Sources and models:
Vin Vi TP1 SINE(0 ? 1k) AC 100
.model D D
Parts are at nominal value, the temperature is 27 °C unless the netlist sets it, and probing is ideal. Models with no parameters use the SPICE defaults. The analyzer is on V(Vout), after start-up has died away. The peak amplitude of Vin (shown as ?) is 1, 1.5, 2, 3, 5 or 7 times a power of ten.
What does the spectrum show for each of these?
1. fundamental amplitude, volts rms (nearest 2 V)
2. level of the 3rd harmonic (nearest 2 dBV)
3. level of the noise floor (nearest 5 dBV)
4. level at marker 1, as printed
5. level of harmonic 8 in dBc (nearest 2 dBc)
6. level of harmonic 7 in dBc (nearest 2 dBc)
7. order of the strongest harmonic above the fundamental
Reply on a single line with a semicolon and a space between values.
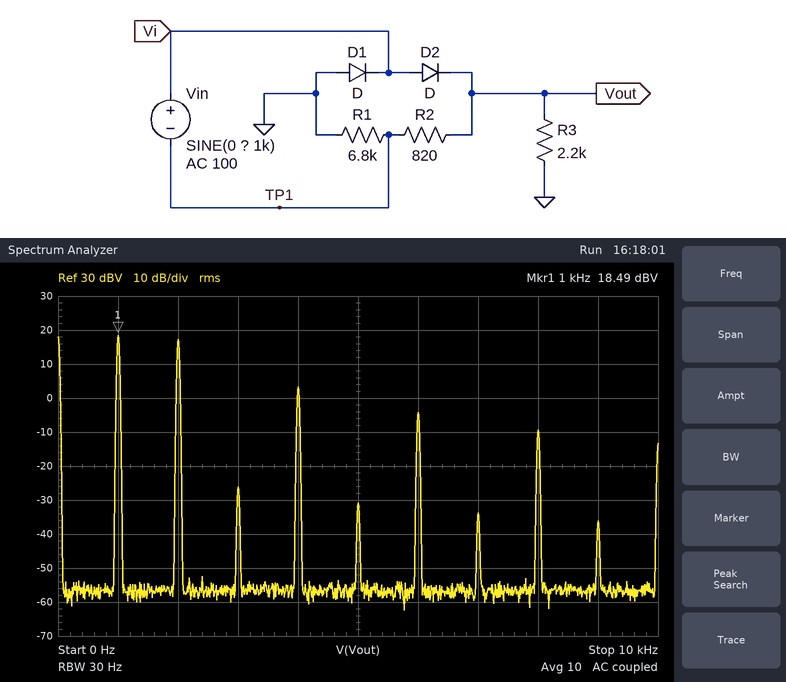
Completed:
8 V; -26 dBV; -55 dBV; 18.49 dBV; -28 dBc; -52 dBc; 2
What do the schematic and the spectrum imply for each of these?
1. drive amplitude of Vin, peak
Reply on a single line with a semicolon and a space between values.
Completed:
50 V
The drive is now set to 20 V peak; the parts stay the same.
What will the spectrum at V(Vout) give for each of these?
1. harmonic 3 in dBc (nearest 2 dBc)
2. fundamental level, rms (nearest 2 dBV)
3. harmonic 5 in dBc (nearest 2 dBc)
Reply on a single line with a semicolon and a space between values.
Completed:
-36 dBc; 10 dBV; -42 dBc
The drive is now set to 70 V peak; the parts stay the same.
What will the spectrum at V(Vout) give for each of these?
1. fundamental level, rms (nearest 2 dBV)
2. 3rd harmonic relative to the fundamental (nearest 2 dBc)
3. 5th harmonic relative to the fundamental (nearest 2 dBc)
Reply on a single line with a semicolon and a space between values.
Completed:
22 dBV; -48 dBc; -52 dBc
